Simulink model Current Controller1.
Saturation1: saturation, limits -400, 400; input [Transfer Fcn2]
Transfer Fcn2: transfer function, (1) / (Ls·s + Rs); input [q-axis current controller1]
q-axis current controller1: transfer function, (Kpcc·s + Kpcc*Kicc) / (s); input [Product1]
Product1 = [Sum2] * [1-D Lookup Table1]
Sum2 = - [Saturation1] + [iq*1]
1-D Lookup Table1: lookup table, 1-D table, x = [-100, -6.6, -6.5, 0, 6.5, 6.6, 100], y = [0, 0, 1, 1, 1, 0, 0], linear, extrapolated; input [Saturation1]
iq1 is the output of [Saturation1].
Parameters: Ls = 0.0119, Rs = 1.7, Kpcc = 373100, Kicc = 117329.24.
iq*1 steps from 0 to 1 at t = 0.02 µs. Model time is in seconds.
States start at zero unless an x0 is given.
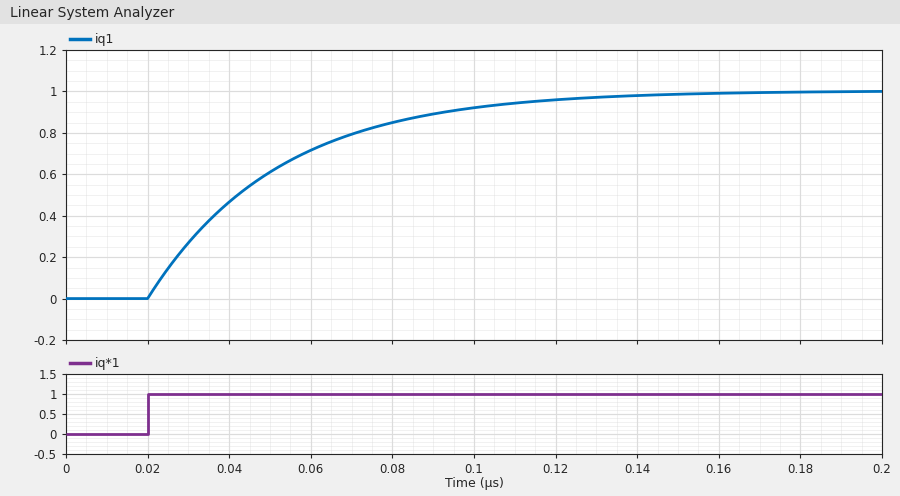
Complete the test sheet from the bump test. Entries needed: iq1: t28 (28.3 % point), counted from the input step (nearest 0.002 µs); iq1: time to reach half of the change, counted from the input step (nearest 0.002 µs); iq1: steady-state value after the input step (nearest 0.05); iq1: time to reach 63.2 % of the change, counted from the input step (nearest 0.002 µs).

0.010 µs
0.022 µs
1.00
0.032 µs
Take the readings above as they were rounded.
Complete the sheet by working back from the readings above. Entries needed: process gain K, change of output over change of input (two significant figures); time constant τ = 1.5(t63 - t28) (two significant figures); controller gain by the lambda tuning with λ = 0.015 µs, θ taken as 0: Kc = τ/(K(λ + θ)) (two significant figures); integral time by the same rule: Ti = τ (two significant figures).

1.0
0.033 µs
2.2
0.033 µs
